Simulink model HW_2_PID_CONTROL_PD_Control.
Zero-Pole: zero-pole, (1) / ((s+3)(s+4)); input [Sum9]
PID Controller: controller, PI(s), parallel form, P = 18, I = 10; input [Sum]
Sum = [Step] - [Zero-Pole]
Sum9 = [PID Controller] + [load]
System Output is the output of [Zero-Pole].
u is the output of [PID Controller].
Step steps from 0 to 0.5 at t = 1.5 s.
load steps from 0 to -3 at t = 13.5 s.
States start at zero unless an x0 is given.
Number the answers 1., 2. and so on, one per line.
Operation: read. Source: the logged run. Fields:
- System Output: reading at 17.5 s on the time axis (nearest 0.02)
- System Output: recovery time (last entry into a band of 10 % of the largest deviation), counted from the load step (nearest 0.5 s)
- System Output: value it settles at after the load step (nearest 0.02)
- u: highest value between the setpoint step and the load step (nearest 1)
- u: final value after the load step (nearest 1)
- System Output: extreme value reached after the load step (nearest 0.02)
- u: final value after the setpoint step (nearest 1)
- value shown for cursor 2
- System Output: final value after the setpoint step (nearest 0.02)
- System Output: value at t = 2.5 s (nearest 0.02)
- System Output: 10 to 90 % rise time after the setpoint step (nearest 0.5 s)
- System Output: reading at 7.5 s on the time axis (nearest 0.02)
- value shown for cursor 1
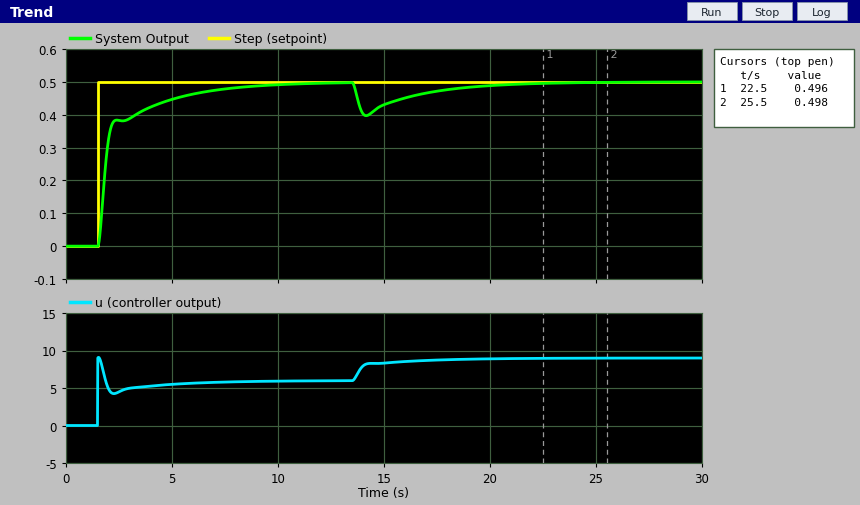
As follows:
1. 0.48
2. 7.0 s
3. 0.50
4. 9
5. 9
6. 0.40
7. 6
8. 0.498
9. 0.50
10. 0.38
11. 3.5 s
12. 0.48
13. 0.496
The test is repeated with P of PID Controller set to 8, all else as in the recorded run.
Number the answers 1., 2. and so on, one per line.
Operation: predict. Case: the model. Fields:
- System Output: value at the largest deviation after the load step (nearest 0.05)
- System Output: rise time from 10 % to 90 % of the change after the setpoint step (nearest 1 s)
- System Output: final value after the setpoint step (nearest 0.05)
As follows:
1. 0.35
2. 3 s
3. 0.50
